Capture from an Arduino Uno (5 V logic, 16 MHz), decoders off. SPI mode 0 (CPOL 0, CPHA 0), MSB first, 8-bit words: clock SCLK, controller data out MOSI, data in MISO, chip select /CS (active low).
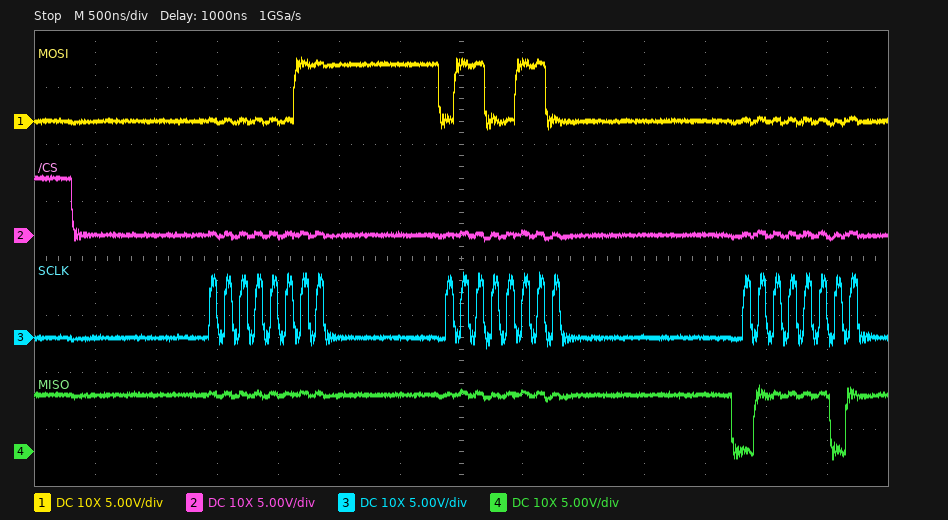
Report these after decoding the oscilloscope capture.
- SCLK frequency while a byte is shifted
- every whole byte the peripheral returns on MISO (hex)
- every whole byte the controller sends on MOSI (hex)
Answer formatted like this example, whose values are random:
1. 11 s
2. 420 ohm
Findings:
1. 8 MHz
2. FF FF 7D
3. 03 66 00
